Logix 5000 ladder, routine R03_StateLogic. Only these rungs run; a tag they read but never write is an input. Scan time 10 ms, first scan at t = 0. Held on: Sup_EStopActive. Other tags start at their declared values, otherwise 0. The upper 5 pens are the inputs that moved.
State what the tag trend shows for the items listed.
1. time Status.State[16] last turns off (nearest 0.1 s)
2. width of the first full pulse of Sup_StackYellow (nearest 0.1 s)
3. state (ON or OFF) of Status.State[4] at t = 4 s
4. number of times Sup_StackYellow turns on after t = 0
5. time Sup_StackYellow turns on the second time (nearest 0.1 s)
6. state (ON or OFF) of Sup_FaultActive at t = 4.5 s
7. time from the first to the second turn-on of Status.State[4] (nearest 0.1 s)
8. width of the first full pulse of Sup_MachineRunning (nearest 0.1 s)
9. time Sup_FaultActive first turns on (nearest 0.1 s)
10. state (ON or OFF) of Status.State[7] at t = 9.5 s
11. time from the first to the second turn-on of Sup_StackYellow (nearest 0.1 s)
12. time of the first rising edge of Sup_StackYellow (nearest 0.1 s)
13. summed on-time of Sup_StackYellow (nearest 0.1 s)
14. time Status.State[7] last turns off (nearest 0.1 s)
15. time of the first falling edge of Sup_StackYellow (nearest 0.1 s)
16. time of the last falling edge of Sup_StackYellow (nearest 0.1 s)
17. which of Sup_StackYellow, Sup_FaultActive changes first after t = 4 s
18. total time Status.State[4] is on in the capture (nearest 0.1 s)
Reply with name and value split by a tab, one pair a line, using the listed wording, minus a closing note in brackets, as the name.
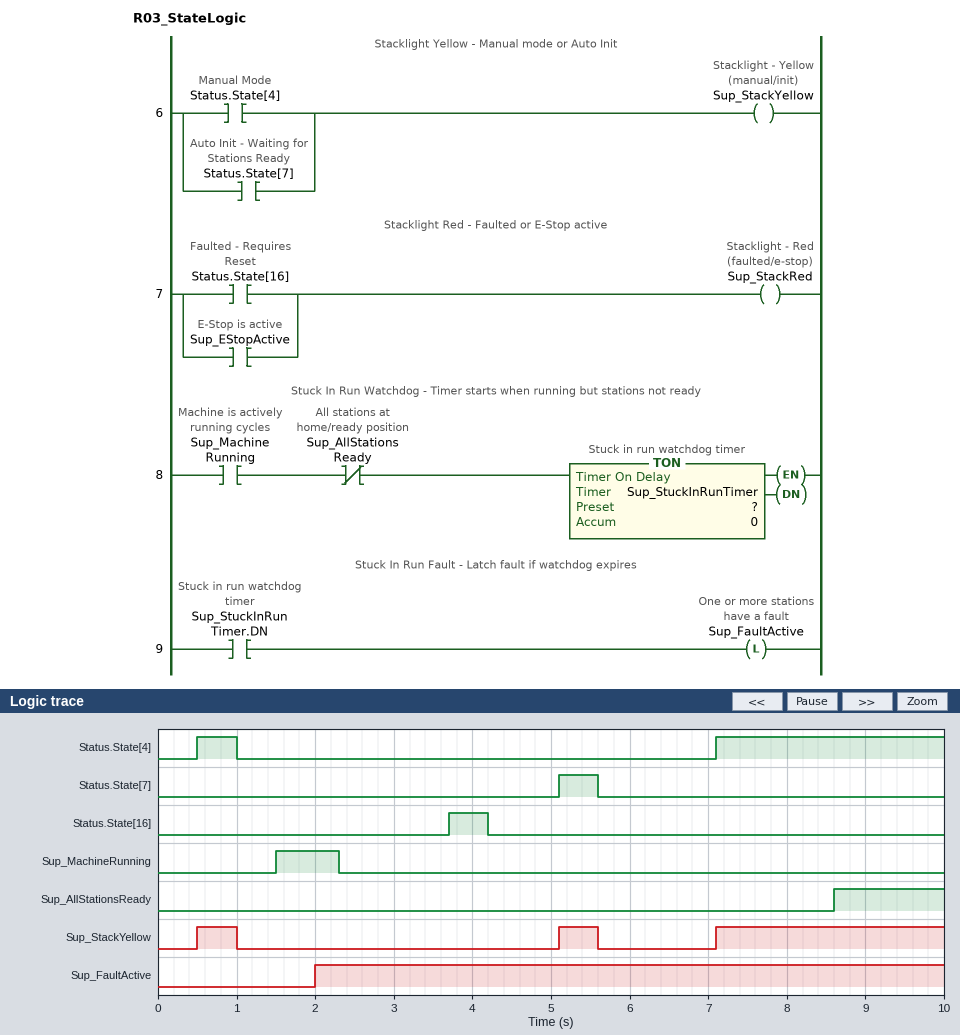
time Status.State[16] last turns off	4.2 s
width of the first full pulse of Sup_StackYellow	0.5 s
state (ON or OFF) of Status.State[4] at t = 4 s	OFF
number of times Sup_StackYellow turns on after t = 0	3
time Sup_StackYellow turns on the second time	5.1 s
state (ON or OFF) of Sup_FaultActive at t = 4.5 s	ON
time from the first to the second turn-on of Status.State[4]	6.6 s
width of the first full pulse of Sup_MachineRunning	0.8 s
time Sup_FaultActive first turns on	2.0 s
state (ON or OFF) of Status.State[7] at t = 9.5 s	OFF
time from the first to the second turn-on of Sup_StackYellow	4.6 s
time of the first rising edge of Sup_StackYellow	0.5 s
summed on-time of Sup_StackYellow	3.9 s
time Status.State[7] last turns off	5.6 s
time of the first falling edge of Sup_StackYellow	1.0 s
time of the last falling edge of Sup_StackYellow	5.6 s
which of Sup_StackYellow, Sup_FaultActive changes first after t = 4 s	Sup_StackYellow
total time Status.State[4] is on in the capture	3.4 s
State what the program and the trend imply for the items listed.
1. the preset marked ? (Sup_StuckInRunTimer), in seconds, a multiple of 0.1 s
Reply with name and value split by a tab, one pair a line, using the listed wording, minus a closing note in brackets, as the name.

the preset marked ? (Sup_StuckInRunTimer), in seconds, a multiple of 0.1 s	0.5 s
